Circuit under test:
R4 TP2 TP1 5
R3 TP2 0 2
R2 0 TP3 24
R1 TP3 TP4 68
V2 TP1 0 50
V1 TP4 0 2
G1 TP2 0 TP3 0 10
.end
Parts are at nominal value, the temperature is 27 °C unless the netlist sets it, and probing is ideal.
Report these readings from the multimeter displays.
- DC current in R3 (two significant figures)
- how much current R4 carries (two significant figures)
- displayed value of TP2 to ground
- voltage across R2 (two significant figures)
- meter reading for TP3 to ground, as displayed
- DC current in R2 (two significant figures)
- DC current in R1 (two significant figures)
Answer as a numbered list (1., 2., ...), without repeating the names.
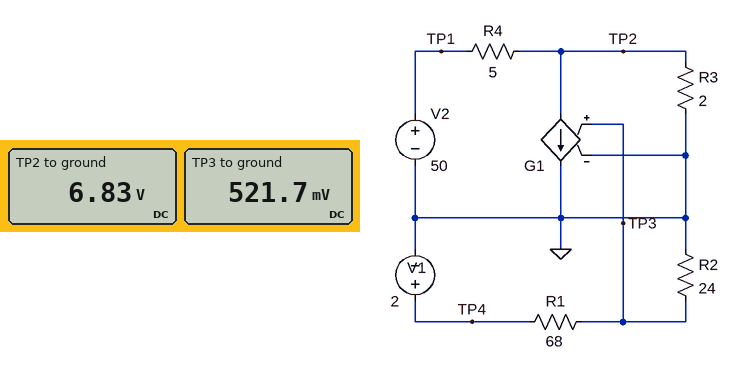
1. 3.4 A
2. 8.6 A
3. 6.83 V
4. 520 mV
5. 521.7 mV
6. 22 mA
7. 22 mA
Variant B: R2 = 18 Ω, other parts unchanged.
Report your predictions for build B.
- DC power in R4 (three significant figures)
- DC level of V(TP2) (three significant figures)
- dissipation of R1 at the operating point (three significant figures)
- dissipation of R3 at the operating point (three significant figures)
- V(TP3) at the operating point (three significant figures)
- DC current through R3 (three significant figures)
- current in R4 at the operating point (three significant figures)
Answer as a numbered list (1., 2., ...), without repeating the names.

1. 348 W
2. 8.31 V
3. 36.8 mW
4. 34.5 W
5. 419 mV
6. 4.15 A
7. 8.34 A
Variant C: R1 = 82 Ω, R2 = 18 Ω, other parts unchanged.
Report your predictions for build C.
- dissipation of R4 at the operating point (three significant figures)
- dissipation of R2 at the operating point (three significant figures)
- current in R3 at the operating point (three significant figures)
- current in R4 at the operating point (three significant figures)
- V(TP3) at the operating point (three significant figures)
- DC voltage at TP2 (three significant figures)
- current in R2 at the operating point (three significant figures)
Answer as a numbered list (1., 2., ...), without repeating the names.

1. 334 W
2. 7.20 mW
3. 4.57 A
4. 8.17 A
5. 360 mV
6. 9.14 V
7. 20.0 mA
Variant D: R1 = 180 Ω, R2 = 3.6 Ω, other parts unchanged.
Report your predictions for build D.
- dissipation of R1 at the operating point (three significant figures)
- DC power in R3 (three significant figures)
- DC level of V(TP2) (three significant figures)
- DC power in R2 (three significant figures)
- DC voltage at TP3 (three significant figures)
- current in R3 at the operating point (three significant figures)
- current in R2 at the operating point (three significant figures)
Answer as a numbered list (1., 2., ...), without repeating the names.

1. 21.4 mW
2. 94.2 W
3. 13.7 V
4. 427 µW
5. 39.2 mV
6. 6.86 A
7. 10.9 mA
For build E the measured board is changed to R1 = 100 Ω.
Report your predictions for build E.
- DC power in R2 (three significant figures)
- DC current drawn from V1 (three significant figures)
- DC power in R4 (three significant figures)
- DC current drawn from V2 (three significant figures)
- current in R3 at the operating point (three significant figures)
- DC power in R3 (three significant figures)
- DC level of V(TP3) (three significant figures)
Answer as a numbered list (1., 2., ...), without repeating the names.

1. 6.24 mW
2. 16.1 mA
3. 340 W
4. 8.25 A
5. 4.38 A
6. 38.3 W
7. 387 mV
